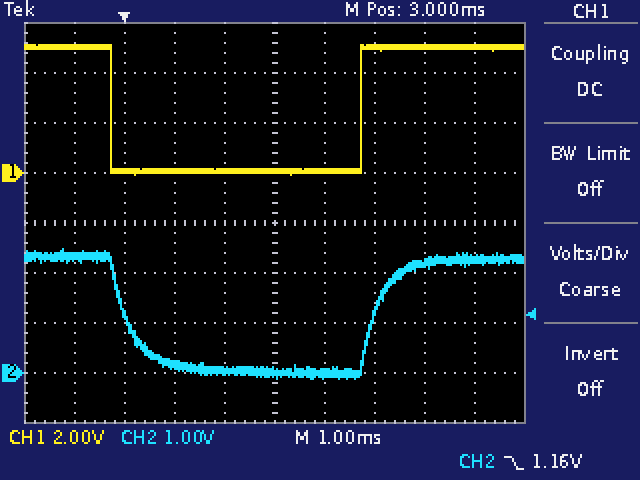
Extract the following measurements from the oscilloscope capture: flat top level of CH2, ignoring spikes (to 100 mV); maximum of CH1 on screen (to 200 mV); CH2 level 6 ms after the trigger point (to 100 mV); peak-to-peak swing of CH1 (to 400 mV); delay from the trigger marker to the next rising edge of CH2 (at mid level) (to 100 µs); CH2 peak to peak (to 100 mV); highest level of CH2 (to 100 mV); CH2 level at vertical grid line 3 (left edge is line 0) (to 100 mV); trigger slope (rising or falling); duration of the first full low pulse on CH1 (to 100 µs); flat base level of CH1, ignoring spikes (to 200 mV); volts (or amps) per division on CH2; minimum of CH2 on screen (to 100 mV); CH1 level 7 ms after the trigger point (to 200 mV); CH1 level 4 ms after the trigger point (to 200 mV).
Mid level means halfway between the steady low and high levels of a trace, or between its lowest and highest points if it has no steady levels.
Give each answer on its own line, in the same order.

2.3 V
5.2 V
2.2 V
5.2 V
5.0 ms
2.6 V
2.5 V
200 mV
falling
5.0 ms
0.0 V
1 V
-100 mV
5.0 V
0.0 V
